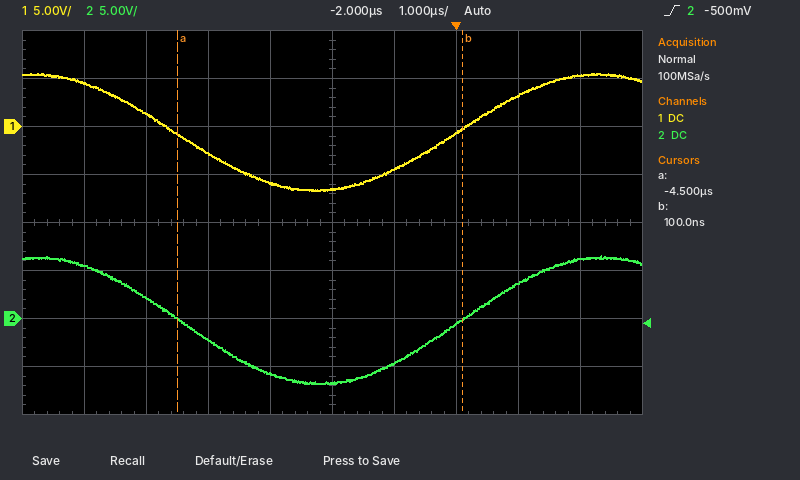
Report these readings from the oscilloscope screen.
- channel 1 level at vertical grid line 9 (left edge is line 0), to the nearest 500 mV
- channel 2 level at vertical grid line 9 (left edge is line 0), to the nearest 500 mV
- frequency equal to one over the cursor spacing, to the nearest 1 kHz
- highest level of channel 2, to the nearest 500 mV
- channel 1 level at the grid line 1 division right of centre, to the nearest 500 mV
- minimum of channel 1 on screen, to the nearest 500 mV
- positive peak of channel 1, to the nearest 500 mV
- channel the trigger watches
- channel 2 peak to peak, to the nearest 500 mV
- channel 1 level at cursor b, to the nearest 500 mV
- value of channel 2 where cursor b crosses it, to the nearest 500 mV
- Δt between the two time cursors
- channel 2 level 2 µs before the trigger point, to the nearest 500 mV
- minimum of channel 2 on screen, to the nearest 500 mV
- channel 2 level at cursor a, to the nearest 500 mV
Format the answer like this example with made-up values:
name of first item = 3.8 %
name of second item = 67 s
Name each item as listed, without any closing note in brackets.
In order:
channel 1 level at vertical grid line 9 (left edge is line 0), to the nearest 500 mV = 5.5 V
channel 2 level at vertical grid line 9 (left edge is line 0), to the nearest 500 mV = 6.0 V
frequency equal to one over the cursor spacing, to the nearest 1 kHz = 217 kHz
highest level of channel 2, to the nearest 500 mV = 6.5 V
channel 1 level at the grid line 1 division right of centre, to the nearest 500 mV = -4.5 V
minimum of channel 1 on screen, to the nearest 500 mV = -6.5 V
positive peak of channel 1, to the nearest 500 mV = 5.5 V
channel the trigger watches = channel 2
channel 2 peak to peak, to the nearest 500 mV = 13.5 V
channel 1 level at cursor b, to the nearest 500 mV = 0.0 V
value of channel 2 where cursor b crosses it, to the nearest 500 mV = 0.0 V
Δt between the two time cursors = 4.6 µs
channel 2 level 2 µs before the trigger point, to the nearest 500 mV = -6.5 V
minimum of channel 2 on screen, to the nearest 500 mV = -7.0 V
channel 2 level at cursor a, to the nearest 500 mV = 0.0 V
